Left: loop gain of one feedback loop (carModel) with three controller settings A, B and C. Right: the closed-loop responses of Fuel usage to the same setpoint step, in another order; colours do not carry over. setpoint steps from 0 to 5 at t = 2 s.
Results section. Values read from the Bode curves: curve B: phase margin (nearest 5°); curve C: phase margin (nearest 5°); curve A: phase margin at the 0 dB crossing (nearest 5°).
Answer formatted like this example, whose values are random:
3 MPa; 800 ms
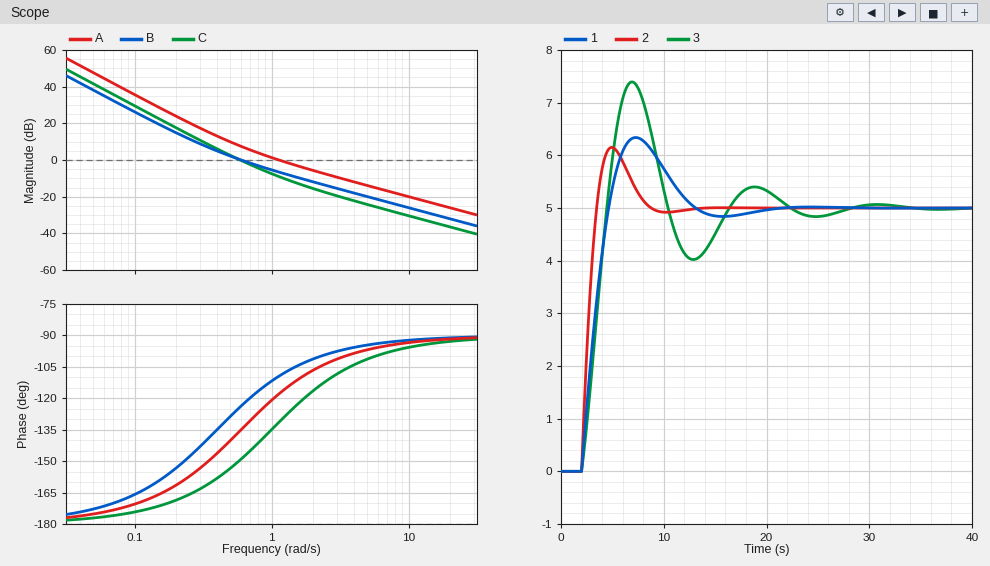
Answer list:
55°; 30°; 60°
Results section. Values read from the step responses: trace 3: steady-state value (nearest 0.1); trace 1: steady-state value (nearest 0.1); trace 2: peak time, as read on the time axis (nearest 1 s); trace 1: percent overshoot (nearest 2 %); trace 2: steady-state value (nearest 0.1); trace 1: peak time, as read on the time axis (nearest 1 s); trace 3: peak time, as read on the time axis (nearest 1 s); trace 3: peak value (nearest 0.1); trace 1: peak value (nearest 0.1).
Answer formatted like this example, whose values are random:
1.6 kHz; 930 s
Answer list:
5.0; 5.0; 5 s; 26 %; 5.0; 7 s; 7 s; 7.4; 6.3
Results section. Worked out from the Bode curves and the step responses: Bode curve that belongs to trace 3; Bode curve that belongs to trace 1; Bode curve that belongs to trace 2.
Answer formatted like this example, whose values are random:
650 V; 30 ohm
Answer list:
C; B; A
